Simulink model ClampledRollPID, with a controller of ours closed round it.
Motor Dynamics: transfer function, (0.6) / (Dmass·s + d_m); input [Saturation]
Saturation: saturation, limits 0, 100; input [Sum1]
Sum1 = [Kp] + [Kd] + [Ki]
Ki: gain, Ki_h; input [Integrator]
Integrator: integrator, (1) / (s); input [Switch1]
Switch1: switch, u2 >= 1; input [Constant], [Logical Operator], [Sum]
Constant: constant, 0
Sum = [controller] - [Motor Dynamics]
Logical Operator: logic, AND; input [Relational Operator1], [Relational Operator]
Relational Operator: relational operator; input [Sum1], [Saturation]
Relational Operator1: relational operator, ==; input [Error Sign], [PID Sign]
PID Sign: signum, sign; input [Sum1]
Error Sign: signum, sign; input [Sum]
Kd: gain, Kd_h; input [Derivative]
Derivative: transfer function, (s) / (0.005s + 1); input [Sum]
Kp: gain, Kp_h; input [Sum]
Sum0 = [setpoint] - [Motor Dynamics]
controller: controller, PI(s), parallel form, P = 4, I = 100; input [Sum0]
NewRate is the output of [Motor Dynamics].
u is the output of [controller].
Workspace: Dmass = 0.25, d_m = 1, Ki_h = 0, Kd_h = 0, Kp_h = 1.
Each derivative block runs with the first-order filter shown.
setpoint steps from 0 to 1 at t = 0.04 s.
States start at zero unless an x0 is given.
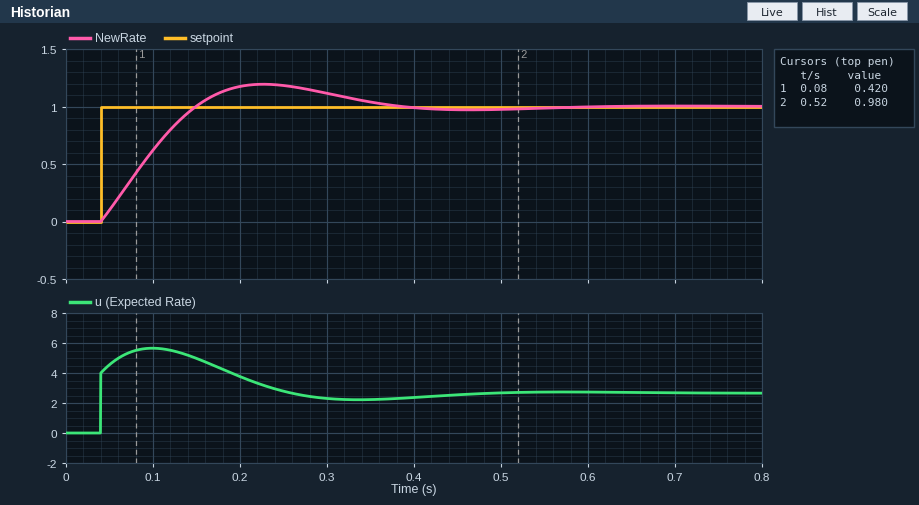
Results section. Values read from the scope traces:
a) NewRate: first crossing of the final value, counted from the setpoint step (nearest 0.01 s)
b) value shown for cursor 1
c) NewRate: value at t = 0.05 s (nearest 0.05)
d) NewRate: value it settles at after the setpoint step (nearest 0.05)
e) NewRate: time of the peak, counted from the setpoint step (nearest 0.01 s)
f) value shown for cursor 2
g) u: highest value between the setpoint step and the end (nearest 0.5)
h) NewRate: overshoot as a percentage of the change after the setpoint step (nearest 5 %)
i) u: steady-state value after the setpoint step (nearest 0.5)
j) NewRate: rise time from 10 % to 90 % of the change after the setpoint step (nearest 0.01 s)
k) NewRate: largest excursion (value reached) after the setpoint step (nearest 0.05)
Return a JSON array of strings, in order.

["0.11 s", "0.420", "0.10", "1.00", "0.19 s", "0.980", "5.5", "20 %", "2.5", "0.08 s", "1.20"]
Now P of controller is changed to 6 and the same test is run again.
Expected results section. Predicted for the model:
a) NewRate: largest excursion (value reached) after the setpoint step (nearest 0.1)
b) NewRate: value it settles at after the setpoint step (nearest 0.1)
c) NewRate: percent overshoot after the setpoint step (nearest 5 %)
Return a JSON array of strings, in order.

["1.1", "1.0", "10 %"]
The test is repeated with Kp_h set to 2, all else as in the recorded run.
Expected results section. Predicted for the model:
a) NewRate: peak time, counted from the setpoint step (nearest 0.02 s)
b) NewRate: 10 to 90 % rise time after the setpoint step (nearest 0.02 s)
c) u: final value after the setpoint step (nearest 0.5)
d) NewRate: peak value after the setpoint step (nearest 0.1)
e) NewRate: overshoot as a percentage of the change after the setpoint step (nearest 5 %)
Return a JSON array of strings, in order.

["0.12 s", "0.06 s", "2.0", "1.1", "15 %"]
